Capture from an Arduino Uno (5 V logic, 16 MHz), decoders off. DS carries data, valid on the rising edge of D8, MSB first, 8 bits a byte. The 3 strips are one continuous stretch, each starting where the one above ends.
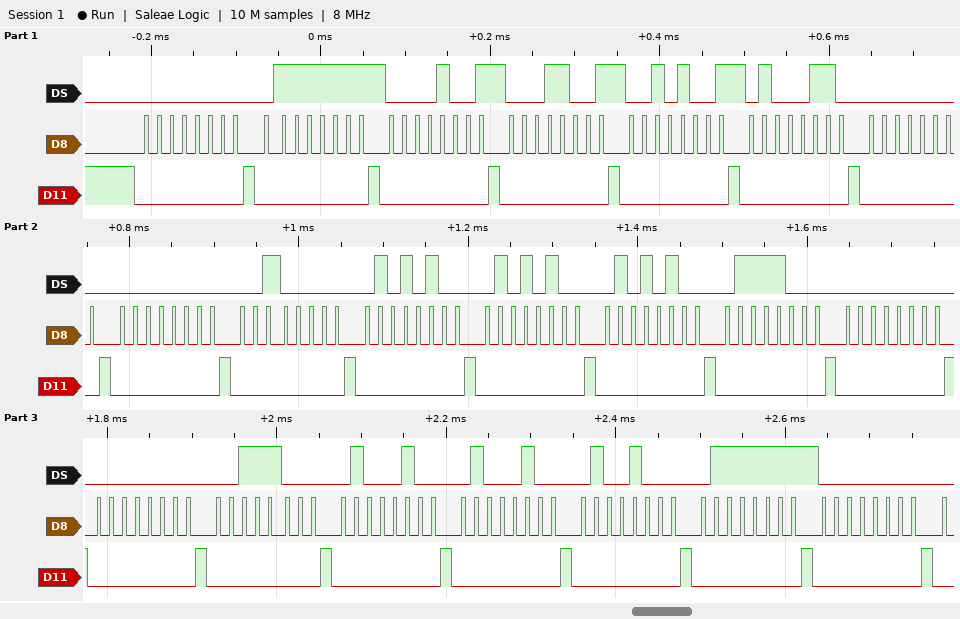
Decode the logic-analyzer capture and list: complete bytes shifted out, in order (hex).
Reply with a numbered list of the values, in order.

1. 00 7F 09 19 29 46 00 00 20 54 54 54 78 00 00 38 44 44 48 7F 00
